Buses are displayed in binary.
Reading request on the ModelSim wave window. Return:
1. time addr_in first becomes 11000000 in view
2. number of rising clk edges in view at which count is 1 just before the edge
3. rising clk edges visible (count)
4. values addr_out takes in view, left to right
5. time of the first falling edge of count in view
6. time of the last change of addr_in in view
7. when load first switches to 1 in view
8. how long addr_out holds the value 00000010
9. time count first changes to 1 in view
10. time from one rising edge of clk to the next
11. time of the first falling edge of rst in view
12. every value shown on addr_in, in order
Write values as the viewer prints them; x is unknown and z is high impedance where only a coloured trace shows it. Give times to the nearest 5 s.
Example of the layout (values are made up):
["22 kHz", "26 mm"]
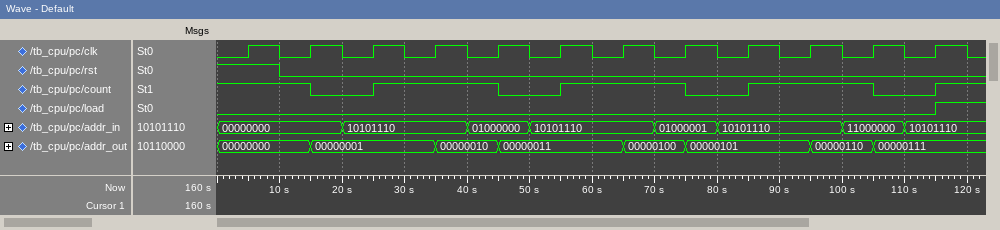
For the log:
["100 s", "8", "12", "00000000, 00000001, 00000010, 00000011, 00000100, 00000101, 00000110, 00000111", "15 s", "110 s", "115 s", "10 s", "25 s", "10 s", "10 s", "00000000, 10101110, 01000000, 10101110, 01000001, 10101110, 11000000, 10101110"]
